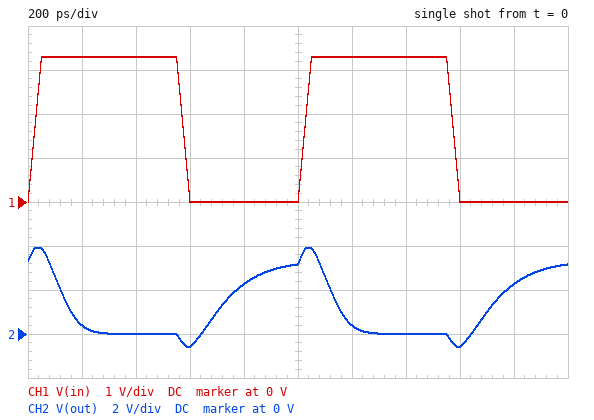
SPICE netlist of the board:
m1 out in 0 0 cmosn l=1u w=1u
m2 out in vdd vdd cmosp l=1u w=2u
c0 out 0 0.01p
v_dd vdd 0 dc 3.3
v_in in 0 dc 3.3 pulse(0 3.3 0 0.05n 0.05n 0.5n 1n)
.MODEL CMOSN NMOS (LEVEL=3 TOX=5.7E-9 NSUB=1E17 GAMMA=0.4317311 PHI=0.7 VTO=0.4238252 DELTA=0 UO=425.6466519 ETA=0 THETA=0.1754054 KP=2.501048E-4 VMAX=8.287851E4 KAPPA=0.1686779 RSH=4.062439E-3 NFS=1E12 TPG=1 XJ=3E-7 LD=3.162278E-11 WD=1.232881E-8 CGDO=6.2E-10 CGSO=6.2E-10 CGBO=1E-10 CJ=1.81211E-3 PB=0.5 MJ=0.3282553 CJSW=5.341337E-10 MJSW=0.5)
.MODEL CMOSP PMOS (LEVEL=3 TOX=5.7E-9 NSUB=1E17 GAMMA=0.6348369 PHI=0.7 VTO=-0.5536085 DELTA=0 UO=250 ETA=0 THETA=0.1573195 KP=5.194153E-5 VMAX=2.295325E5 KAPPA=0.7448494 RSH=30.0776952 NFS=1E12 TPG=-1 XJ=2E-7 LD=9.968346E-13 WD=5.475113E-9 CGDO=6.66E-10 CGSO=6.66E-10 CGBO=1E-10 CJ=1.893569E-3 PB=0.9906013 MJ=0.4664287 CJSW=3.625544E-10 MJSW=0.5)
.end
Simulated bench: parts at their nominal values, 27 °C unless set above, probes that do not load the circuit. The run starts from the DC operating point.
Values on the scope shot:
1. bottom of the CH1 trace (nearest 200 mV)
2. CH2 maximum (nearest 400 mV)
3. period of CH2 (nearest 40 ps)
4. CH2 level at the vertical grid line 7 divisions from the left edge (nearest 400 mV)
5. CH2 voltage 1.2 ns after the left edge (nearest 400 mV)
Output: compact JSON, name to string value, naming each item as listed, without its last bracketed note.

{"bottom of the CH1 trace": "0 V", "CH2 maximum": "4.0 V", "period of CH2": "1.00 ns", "CH2 level at the vertical grid line 7 divisions from the left edge": "0 V", "CH2 voltage 1.2 ns after the left edge": "400 mV"}
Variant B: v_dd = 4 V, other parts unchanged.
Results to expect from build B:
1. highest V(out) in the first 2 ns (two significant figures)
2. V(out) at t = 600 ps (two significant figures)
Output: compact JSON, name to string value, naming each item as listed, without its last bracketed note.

{"highest V(out) in the first 2 ns": "4.6 V", "V(out) at t = 600 ps": "-560 mV"}
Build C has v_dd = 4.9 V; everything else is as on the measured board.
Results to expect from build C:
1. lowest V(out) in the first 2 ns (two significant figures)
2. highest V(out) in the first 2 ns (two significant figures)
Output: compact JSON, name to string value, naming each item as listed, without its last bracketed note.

{"lowest V(out) in the first 2 ns": "-270 mV", "highest V(out) in the first 2 ns": "5.5 V"}
